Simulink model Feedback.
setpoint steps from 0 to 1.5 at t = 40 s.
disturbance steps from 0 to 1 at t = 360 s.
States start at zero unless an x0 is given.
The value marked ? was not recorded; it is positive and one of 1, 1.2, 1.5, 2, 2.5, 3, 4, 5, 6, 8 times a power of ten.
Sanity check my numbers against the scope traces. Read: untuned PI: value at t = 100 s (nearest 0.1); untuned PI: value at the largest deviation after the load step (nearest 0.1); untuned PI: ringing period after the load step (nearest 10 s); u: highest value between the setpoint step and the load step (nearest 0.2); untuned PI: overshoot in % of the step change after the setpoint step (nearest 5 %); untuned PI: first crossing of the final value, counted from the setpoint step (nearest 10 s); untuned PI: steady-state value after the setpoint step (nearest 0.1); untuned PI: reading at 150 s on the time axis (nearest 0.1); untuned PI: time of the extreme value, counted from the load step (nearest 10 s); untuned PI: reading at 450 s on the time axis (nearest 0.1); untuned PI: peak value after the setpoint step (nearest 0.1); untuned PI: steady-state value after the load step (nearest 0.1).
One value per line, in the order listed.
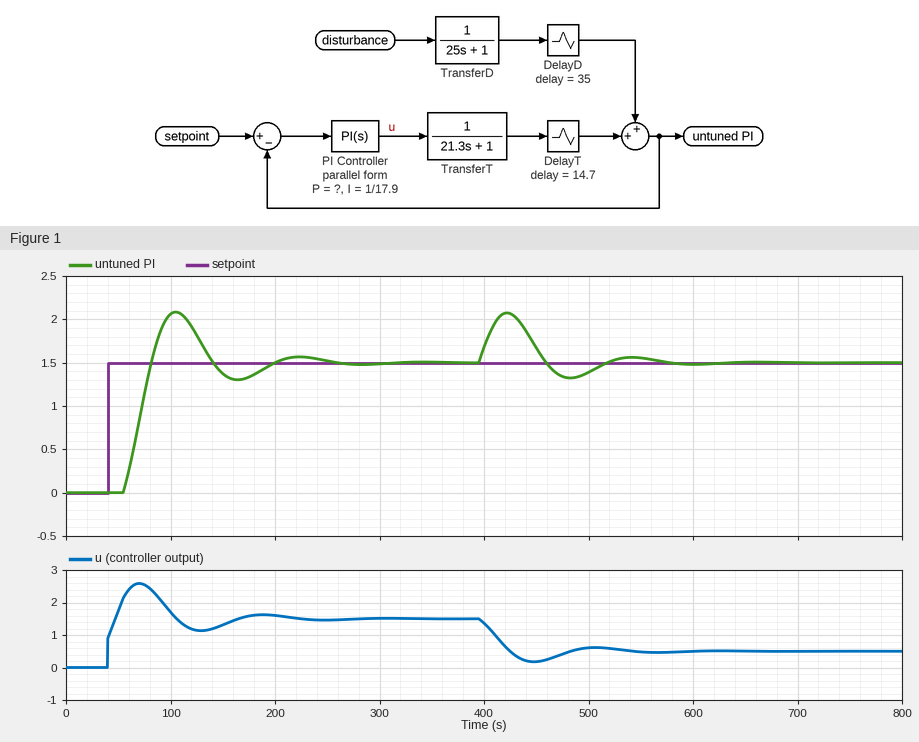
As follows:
2.1
2.1
120 s
2.6
40 %
40 s
1.5
1.4
60 s
1.7
2.1
1.5
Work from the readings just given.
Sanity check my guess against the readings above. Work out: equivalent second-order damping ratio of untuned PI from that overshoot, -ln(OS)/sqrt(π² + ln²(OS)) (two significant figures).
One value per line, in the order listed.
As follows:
0.28
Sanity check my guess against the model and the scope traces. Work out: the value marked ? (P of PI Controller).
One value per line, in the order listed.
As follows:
0.6
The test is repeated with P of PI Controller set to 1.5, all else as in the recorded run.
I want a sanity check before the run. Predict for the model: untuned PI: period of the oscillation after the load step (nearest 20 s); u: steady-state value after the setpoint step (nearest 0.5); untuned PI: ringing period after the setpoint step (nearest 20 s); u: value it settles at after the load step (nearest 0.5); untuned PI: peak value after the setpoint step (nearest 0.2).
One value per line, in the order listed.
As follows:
60 s
1.5
60 s
0.5
2.0
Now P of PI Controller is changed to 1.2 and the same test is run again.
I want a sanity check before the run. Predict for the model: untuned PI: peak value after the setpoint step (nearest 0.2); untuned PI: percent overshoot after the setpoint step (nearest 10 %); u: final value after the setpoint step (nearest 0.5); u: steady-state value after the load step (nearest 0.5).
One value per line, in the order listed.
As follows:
2.0
30 %
1.5
0.5
